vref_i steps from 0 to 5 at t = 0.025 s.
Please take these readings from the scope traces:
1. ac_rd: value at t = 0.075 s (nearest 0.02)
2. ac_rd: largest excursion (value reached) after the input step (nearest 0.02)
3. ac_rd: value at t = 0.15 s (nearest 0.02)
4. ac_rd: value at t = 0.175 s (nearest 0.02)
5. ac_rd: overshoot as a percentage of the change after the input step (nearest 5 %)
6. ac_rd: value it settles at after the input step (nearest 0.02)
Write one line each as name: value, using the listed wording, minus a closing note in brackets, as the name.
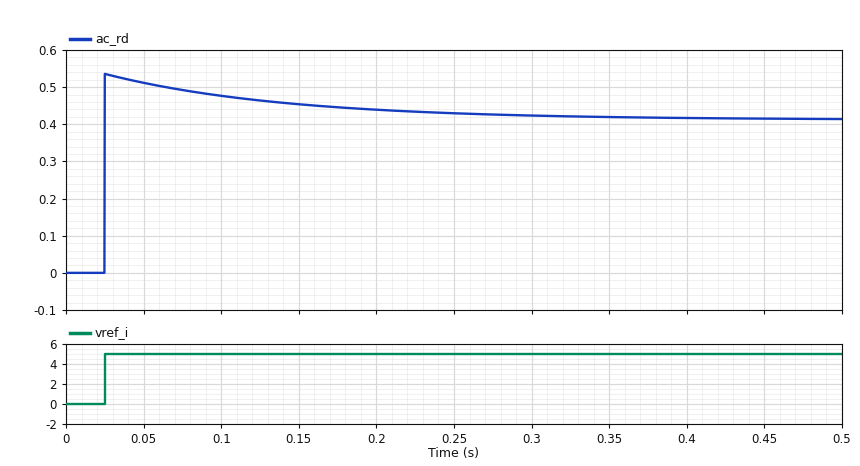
ac_rd: value at t = 0.075 s: 0.50
ac_rd: largest excursion (value reached) after the input step: 0.54
ac_rd: value at t = 0.15 s: 0.46
ac_rd: value at t = 0.175 s: 0.44
ac_rd: overshoot as a percentage of the change after the input step: 30 %
ac_rd: value it settles at after the input step: 0.42
